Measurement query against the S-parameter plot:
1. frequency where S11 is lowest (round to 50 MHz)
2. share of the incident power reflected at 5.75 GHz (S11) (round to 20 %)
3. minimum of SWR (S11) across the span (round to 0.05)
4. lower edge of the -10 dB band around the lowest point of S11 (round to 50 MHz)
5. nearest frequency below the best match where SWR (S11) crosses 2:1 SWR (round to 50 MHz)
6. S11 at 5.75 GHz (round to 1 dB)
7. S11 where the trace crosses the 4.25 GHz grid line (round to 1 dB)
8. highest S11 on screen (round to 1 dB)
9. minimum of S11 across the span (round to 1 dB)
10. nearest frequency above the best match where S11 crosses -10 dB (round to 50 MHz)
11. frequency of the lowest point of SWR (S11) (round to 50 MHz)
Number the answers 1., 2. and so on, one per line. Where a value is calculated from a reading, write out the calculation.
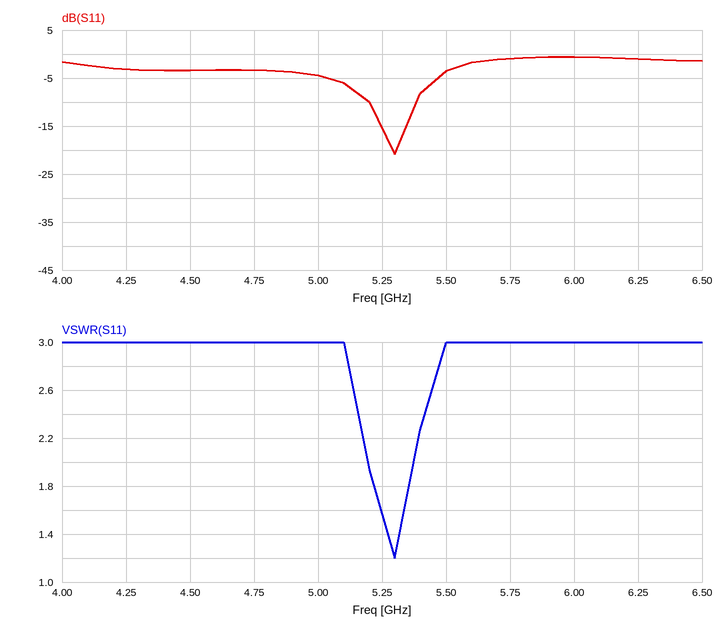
1. 5.30 GHz
2. 10^(-1/10) ≈ 79.4 %, so 80 % to the nearest 20 %
3. 1.20
4. 5.20 GHz
5. 5.20 GHz
6. -1 dB
7. -3 dB
8. -1 dB
9. -21 dB
10. 5.40 GHz
11. 5.30 GHz
